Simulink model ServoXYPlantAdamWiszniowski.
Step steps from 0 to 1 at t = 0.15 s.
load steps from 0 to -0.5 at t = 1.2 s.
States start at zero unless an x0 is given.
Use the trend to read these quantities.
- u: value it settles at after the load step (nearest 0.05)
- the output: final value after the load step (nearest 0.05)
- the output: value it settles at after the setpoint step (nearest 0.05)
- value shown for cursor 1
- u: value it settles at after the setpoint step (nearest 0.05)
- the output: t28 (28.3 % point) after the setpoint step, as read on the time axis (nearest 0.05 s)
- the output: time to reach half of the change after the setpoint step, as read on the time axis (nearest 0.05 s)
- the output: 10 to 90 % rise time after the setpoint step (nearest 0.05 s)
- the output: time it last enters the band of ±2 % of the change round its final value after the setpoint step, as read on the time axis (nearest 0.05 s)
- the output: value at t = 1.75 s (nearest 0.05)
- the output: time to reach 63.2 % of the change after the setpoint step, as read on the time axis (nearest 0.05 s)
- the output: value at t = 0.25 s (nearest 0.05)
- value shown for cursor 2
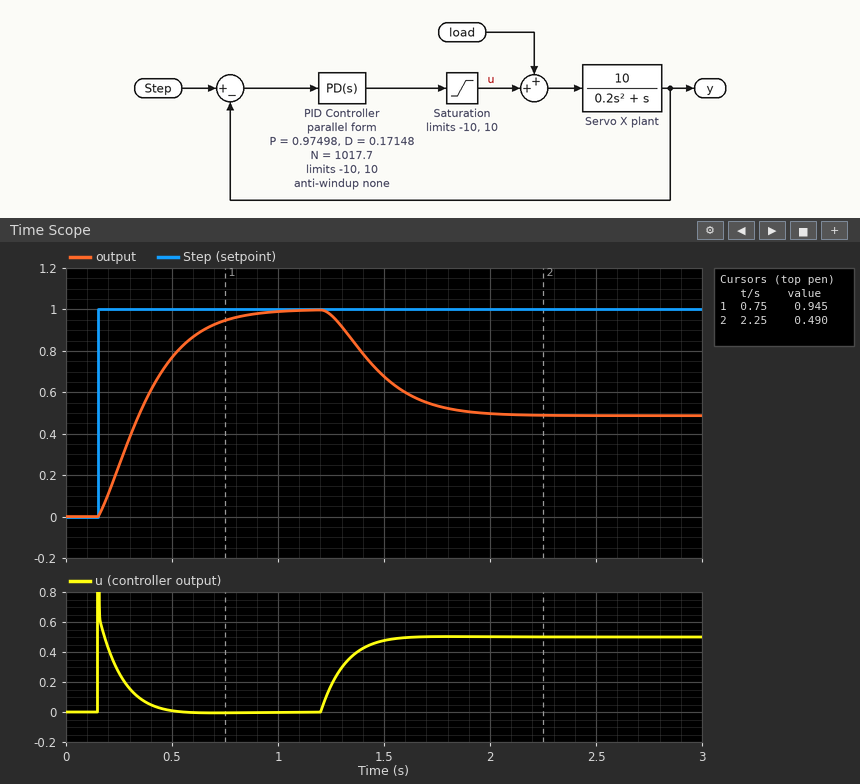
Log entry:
0.50
0.50
1.00
0.945
0.00
0.25 s
0.35 s
0.45 s
0.90 s
0.55
0.40 s
0.25
0.490
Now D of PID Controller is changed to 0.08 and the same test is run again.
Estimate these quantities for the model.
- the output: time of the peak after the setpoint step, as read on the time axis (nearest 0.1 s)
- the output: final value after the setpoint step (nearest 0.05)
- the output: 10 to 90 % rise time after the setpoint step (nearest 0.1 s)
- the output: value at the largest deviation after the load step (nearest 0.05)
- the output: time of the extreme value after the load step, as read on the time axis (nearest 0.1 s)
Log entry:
0.7 s
1.00
0.3 s
0.45
1.8 s
